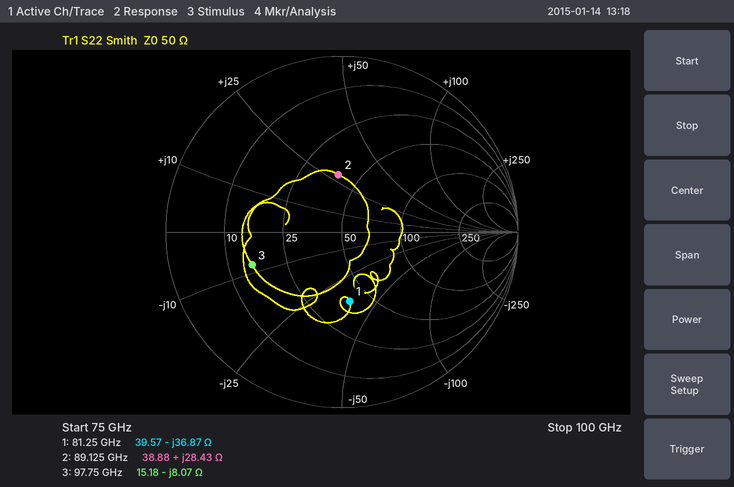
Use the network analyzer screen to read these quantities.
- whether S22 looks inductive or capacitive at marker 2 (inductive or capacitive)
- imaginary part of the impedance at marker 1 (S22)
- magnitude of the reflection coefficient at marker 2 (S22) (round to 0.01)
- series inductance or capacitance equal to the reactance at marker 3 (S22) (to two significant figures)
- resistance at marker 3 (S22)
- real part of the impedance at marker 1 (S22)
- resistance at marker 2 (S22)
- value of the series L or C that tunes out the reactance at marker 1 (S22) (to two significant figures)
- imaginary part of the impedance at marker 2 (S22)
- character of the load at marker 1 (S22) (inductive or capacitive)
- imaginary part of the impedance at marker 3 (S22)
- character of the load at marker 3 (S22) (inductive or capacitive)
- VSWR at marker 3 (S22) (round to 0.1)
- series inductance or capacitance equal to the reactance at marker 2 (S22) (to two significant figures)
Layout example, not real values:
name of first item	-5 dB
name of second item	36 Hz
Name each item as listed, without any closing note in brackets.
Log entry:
whether S22 looks inductive or capacitive at marker 2	inductive
imaginary part of the impedance at marker 1	-36.87 Ω
magnitude of the reflection coefficient at marker 2 (S22)	0.33
series inductance or capacitance equal to the reactance at marker 3 (S22)	200 fF
resistance at marker 3	15.18 Ω
real part of the impedance at marker 1	39.57 Ω
resistance at marker 2	38.88 Ω
value of the series L or C that tunes out the reactance at marker 1 (S22)	72 pH
imaginary part of the impedance at marker 2	+28.43 Ω
character of the load at marker 1 (S22)	capacitive
imaginary part of the impedance at marker 3	-8.07 Ω
character of the load at marker 3 (S22)	capacitive
VSWR at marker 3 (S22)	3.4
series inductance or capacitance equal to the reactance at marker 2 (S22)	51 pH
